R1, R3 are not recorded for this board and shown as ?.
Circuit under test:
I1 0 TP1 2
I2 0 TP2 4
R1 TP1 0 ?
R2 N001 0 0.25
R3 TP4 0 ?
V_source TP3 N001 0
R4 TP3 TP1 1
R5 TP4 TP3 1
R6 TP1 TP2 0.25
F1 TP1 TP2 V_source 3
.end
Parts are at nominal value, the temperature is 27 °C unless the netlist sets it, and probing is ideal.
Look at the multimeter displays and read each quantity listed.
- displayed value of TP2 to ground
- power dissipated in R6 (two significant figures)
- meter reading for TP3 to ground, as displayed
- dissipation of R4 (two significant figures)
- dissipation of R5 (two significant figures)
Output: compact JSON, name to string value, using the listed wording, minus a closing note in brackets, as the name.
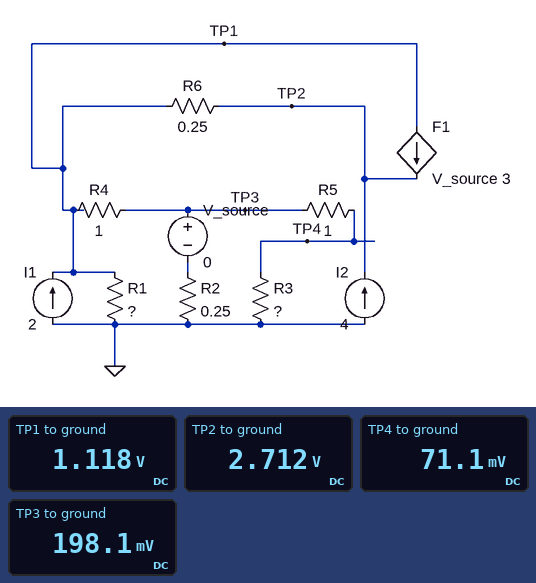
{"displayed value of TP2 to ground": "2.712 V", "power dissipated in R6": "10 W", "meter reading for TP3 to ground, as displayed": "198.1 mV", "dissipation of R4": "850 mW", "dissipation of R5": "16 mW"}
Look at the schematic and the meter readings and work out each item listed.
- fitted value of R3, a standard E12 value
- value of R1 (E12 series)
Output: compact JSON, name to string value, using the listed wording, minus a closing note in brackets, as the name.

{"fitted value of R3, a standard E12 value": "0.56 Ω", "value of R1": "0.22 Ω"}
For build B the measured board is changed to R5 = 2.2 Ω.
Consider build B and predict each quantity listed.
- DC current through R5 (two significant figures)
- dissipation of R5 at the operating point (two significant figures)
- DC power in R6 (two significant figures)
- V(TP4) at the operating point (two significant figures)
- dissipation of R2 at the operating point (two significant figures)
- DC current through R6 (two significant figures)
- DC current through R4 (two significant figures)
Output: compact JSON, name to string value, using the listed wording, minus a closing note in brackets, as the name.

{"DC current through R5": "76 mA", "dissipation of R5 at the operating point": "13 mW", "DC power in R6": "11 W", "V(TP4) at the operating point": "42 mV", "dissipation of R2 at the operating point": "170 mW", "DC current through R6": "6.5 A", "DC current through R4": "910 mA"}
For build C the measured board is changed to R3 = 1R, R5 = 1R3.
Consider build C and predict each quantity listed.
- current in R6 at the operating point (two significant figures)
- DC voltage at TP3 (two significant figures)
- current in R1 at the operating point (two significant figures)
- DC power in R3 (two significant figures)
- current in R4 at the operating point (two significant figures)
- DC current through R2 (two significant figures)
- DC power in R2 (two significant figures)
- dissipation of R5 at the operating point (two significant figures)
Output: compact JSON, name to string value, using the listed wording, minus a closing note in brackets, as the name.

{"current in R6 at the operating point": "6.5 A", "DC voltage at TP3": "210 mV", "current in R1 at the operating point": "5.1 A", "DC power in R3": "8.0 mW", "current in R4 at the operating point": "910 mA", "DC current through R2": "820 mA", "DC power in R2": "170 mW", "dissipation of R5 at the operating point": "10 mW"}
